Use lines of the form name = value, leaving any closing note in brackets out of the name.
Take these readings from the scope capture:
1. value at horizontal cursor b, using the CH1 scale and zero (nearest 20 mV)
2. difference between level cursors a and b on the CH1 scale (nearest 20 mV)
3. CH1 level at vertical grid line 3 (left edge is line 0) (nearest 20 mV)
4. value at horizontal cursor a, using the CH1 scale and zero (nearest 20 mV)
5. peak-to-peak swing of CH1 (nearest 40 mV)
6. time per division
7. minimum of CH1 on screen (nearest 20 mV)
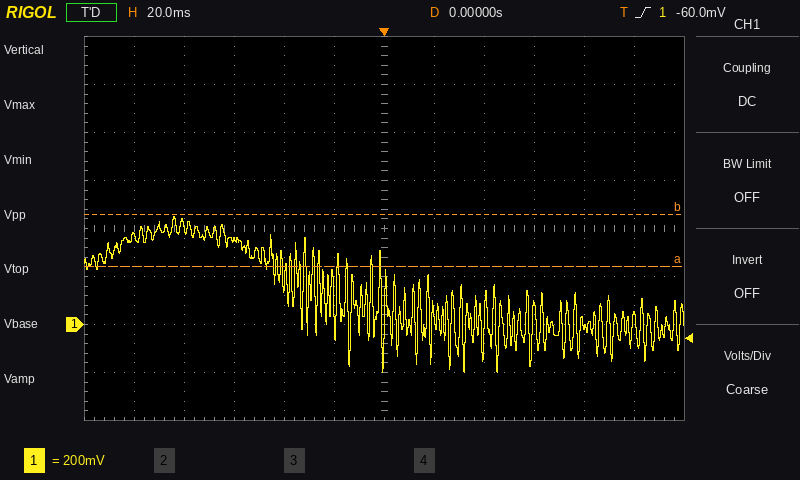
value at horizontal cursor b, using the CH1 scale and zero = 460 mV
difference between level cursors a and b on the CH1 scale = 220 mV
CH1 level at vertical grid line 3 (left edge is line 0) = 360 mV
value at horizontal cursor a, using the CH1 scale and zero = 240 mV
peak-to-peak swing of CH1 = 640 mV
time per division = 20 ms
minimum of CH1 on screen = -200 mV
